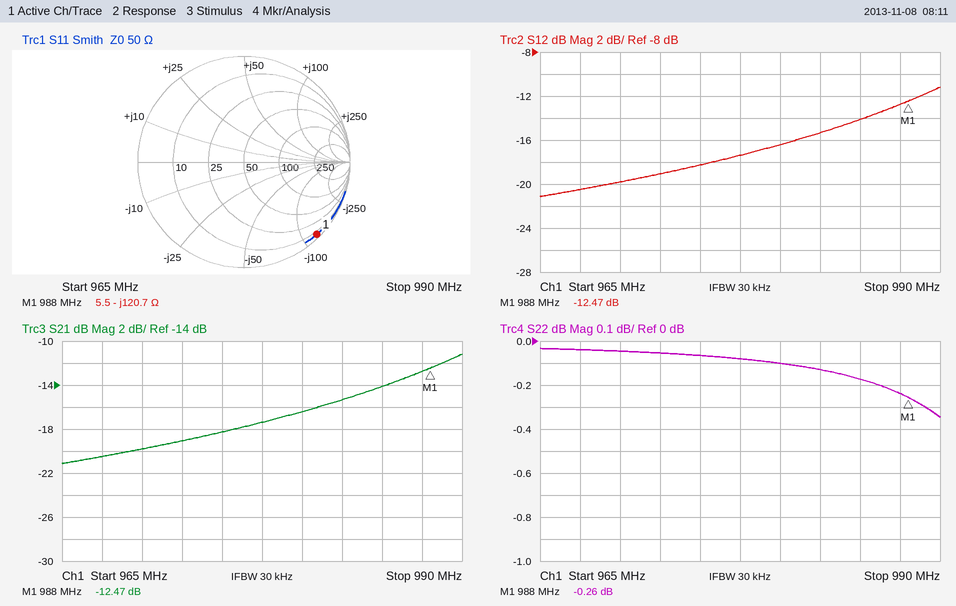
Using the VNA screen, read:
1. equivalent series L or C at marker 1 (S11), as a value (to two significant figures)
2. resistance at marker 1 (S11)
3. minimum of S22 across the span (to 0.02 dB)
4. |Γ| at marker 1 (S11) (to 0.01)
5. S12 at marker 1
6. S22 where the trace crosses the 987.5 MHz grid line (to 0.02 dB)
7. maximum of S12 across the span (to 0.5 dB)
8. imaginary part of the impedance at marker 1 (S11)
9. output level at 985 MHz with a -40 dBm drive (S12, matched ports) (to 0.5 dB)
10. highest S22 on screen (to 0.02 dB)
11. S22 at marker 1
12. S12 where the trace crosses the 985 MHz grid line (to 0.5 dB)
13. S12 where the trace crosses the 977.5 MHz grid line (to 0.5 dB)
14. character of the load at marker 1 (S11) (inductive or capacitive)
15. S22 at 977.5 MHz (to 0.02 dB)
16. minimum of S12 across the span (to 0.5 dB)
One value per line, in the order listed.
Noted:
1.3 pF
5.5 Ω
-0.34 dB
0.97
-12.47 dB
-0.24 dB
-11.0 dB
-120.7 Ω
-54.0 dBm
-0.04 dB
-0.26 dB
-14.0 dB
-17.5 dB
capacitive
-0.08 dB
-21.0 dB
